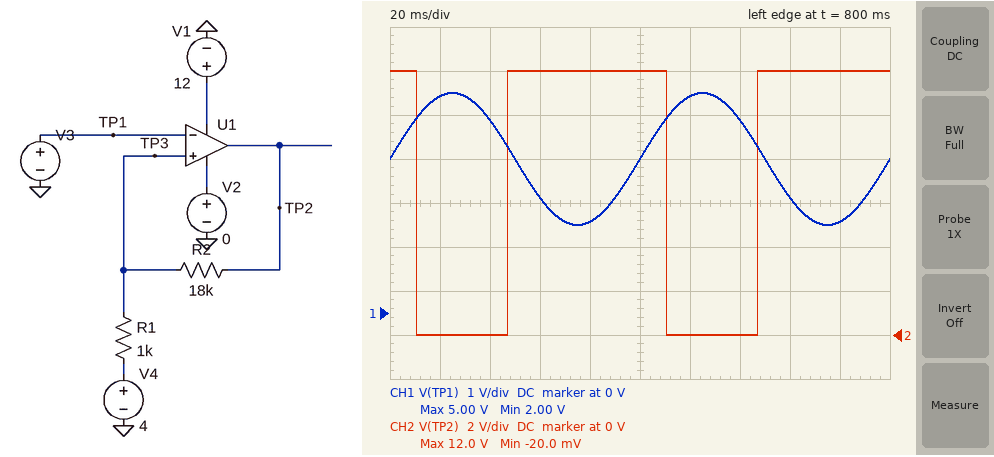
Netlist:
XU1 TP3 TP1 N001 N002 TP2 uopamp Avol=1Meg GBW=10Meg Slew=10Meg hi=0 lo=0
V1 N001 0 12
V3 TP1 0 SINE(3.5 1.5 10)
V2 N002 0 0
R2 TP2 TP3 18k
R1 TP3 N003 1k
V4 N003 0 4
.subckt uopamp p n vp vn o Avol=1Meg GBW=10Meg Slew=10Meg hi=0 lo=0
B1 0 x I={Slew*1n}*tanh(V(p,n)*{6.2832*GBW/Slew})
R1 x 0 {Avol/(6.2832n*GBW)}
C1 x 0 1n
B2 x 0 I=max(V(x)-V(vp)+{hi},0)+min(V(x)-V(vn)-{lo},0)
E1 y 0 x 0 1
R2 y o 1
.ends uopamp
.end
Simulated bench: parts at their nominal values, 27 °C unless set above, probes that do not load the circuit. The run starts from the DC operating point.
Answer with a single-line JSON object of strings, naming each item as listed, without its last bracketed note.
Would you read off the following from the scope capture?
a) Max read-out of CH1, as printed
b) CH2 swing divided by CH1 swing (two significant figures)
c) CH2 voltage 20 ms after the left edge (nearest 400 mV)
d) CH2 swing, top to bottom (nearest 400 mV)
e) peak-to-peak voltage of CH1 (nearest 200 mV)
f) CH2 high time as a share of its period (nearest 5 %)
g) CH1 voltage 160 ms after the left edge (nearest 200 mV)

{"Max read-out of CH1, as printed": "5.00 V", "CH2 swing divided by CH1 swing": "4.0", "CH2 voltage 20 ms after the left edge": "0 V", "CH2 swing, top to bottom": "12.0 V", "peak-to-peak voltage of CH1": "3.0 V", "CH2 high time as a share of its period": "65 %", "CH1 voltage 160 ms after the left edge": "2.6 V"}
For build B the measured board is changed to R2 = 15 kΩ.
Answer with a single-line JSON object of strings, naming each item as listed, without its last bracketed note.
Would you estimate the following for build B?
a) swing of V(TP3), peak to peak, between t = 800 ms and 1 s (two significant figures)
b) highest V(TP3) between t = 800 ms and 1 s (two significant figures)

{"swing of V(TP3), peak to peak, between t = 800 ms and 1 s": "750 mV", "highest V(TP3) between t = 800 ms and 1 s": "4.5 V"}
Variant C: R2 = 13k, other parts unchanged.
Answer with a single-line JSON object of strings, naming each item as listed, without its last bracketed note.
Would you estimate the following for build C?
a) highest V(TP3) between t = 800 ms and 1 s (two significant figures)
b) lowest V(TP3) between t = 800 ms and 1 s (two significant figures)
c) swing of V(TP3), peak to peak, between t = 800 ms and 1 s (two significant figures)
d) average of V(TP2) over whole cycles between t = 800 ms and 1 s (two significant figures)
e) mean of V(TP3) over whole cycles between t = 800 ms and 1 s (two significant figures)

{"highest V(TP3) between t = 800 ms and 1 s": "4.6 V", "lowest V(TP3) between t = 800 ms and 1 s": "3.7 V", "swing of V(TP3), peak to peak, between t = 800 ms and 1 s": "860 mV", "average of V(TP2) over whole cycles between t = 800 ms and 1 s": "7.8 V", "mean of V(TP3) over whole cycles between t = 800 ms and 1 s": "4.3 V"}
